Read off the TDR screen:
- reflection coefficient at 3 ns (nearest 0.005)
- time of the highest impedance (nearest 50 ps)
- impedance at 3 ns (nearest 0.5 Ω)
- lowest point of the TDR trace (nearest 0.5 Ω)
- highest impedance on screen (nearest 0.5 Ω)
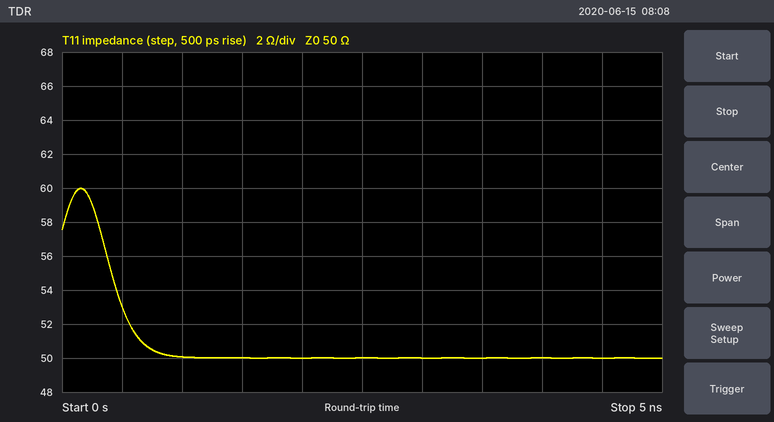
0.000
150 ps
50.0 Ω
50.0 Ω
60.0 Ω
